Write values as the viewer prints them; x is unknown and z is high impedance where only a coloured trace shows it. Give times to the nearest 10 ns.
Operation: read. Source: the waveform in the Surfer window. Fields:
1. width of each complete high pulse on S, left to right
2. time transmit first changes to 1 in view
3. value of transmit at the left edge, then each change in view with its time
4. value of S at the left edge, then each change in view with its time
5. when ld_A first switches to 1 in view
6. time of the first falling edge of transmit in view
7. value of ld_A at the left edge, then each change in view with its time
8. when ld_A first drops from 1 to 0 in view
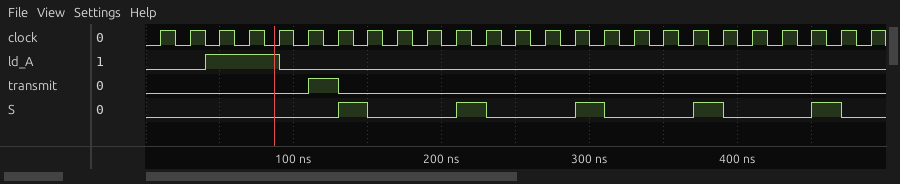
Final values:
20 ns, 20 ns, 20 ns, 20 ns, 20 ns
110 ns
0, 1 at 110 ns, 0 at 130 ns
0, 1 at 130 ns, 0 at 150 ns, 1 at 210 ns, 0 at 230 ns, 1 at 290 ns, 0 at 310 ns, 1 at 370 ns, 0 at 390 ns, 1 at 450 ns, 0 at 470 ns
40 ns
130 ns
0, 1 at 40 ns, 0 at 90 ns
90 ns
